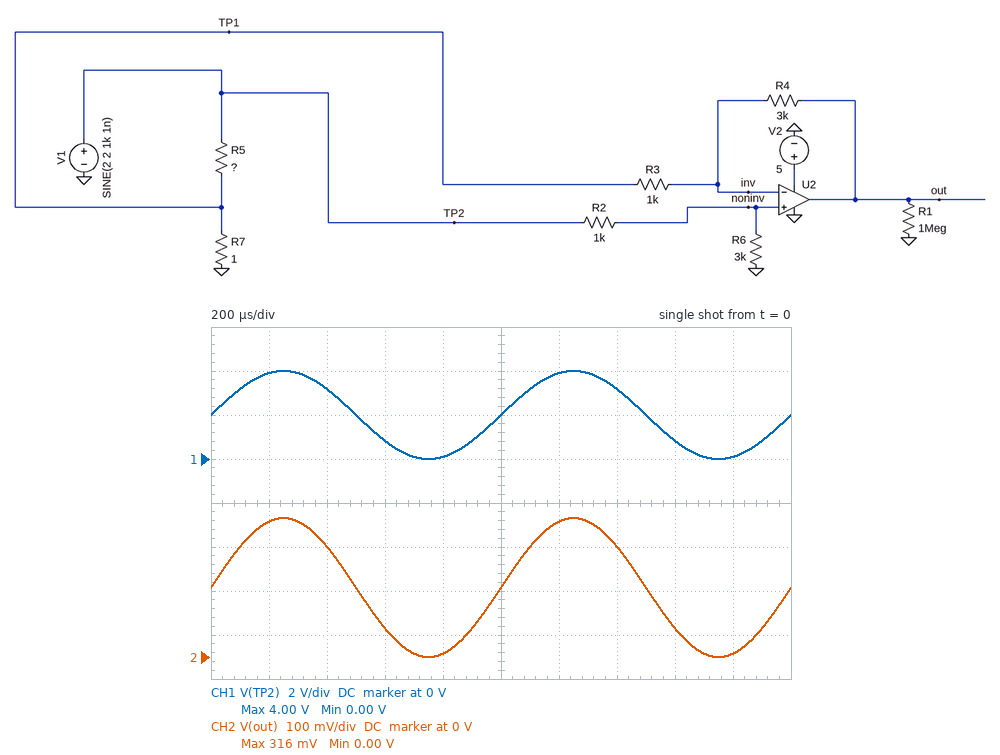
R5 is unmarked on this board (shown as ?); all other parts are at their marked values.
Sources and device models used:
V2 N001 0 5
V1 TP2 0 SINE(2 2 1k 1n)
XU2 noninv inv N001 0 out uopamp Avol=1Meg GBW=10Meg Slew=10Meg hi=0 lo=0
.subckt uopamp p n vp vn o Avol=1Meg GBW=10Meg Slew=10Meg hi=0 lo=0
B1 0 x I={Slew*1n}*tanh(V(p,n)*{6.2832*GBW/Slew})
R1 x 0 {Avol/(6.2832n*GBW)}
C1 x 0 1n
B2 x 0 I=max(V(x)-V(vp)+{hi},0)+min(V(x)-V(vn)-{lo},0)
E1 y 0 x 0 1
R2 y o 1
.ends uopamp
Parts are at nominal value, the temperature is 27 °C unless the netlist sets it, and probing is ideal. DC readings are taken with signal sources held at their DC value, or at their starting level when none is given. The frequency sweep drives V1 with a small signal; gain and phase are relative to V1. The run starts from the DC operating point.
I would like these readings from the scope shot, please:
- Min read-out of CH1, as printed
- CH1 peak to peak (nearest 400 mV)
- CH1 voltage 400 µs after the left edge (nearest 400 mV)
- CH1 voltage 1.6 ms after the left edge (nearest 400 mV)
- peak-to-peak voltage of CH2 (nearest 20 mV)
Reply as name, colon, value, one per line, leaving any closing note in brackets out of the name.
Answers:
Min read-out of CH1, as printed: 0.00 V
CH1 peak to peak: 4.0 V
CH1 voltage 400 µs after the left edge: 3.2 V
CH1 voltage 1.6 ms after the left edge: 800 mV
peak-to-peak voltage of CH2: 320 mV
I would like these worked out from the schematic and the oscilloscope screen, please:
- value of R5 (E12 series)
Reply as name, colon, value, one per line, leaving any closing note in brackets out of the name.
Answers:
value of R5: 0.027 Ω
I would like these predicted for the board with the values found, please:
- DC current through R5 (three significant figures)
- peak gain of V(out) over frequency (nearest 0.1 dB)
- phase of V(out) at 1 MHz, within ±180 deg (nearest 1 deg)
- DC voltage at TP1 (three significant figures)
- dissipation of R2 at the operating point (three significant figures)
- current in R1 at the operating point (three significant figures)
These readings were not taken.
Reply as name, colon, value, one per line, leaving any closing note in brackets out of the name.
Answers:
DC current through R5: 1.95 A
peak gain of V(out) over frequency: -22.1 dB
phase of V(out) at 1 MHz, within ±180 deg: -22 deg
DC voltage at TP1: 1.95 V
dissipation of R2 at the operating point: 250 µW
current in R1 at the operating point: 158 nA
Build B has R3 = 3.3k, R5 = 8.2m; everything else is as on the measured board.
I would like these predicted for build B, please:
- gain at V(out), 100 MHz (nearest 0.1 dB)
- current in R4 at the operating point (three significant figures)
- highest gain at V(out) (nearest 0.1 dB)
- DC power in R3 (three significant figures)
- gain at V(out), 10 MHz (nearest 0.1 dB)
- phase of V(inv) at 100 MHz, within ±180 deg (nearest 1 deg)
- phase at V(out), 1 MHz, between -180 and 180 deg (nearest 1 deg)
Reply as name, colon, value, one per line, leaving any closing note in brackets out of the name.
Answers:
gain at V(out), 100 MHz: -31.1 dB
current in R4 at the operating point: 147 µA
highest gain at V(out): -5.5 dB
DC power in R3: 70.9 µW
gain at V(out), 10 MHz: -12.2 dB
phase of V(inv) at 100 MHz, within ±180 deg: -2 deg
phase at V(out), 1 MHz, between -180 and 180 deg: -11 deg
